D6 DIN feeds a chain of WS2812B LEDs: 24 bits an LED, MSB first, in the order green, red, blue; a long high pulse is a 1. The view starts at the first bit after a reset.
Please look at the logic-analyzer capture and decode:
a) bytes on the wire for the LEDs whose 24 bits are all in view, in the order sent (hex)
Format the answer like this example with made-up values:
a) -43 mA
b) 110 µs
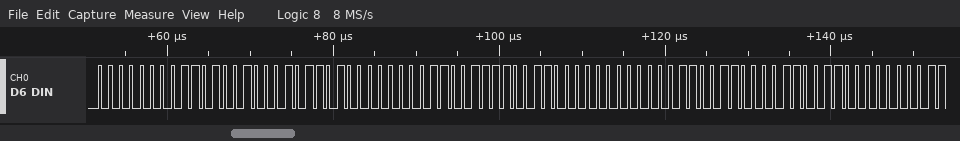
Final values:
a) 00 D2 2D 00 CF 30 00 CC 33
